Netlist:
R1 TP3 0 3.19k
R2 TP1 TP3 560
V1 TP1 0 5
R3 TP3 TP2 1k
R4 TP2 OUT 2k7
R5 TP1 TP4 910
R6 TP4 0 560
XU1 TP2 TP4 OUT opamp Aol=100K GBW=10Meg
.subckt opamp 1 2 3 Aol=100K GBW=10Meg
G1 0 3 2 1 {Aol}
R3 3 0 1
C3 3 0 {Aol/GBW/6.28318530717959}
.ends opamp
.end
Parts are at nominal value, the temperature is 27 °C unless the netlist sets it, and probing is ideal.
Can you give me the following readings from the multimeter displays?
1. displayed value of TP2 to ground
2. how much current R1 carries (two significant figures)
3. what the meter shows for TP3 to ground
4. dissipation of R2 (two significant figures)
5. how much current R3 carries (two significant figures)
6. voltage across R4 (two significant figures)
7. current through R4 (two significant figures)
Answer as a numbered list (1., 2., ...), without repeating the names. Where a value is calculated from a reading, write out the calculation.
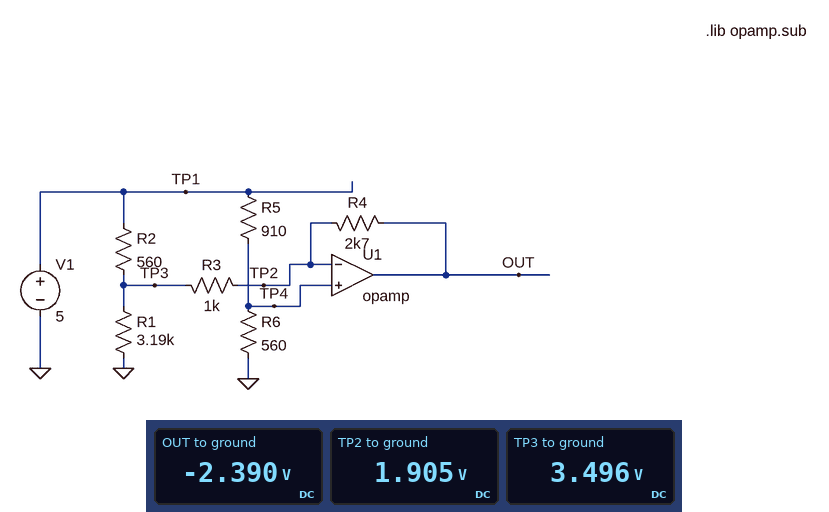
1. 1.905 V
2. (3.496 V) / 3.19 kΩ = 1.1 mA
3. 3.496 V
4. (5 V - 3.496 V)^2 / 560 Ω = 4.0 mW
5. (3.496 V - 1.905 V) / 1 kΩ = 1.6 mA
6. 1.905 V - (-2.39 V) = 4.3 V
7. (1.905 V - (-2.39 V)) / 2.7 kΩ = 1.6 mA
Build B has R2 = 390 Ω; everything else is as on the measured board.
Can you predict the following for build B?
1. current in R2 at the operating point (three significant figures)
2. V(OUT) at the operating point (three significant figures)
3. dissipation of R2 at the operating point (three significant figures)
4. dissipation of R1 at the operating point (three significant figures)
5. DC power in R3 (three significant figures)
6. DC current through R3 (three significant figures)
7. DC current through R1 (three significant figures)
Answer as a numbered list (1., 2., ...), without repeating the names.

1. 3.08 mA
2. -3.21 V
3. 3.71 mW
4. 4.52 mW
5. 3.58 mW
6. 1.89 mA
7. 1.19 mA
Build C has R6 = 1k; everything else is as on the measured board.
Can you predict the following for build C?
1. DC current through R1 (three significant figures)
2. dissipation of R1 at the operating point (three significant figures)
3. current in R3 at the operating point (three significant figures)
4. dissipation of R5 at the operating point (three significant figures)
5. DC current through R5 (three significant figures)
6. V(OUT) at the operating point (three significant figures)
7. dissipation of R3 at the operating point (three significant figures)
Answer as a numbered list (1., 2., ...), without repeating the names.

1. 1.17 mA
2. 4.35 mW
3. 1.11 mA
4. 6.24 mW
5. 2.62 mA
6. -373 mV
7. 1.23 mW
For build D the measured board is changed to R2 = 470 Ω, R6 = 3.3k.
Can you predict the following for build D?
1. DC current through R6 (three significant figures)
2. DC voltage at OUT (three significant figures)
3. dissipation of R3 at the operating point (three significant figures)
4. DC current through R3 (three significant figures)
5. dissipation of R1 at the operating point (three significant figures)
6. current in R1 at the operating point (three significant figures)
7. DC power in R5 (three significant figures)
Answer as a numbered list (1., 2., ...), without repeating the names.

1. 1.19 mA
2. 3.08 V
3. 96.9 µW
4. 311 µA
5. 5.61 mW
6. 1.33 mA
7. 1.28 mW
